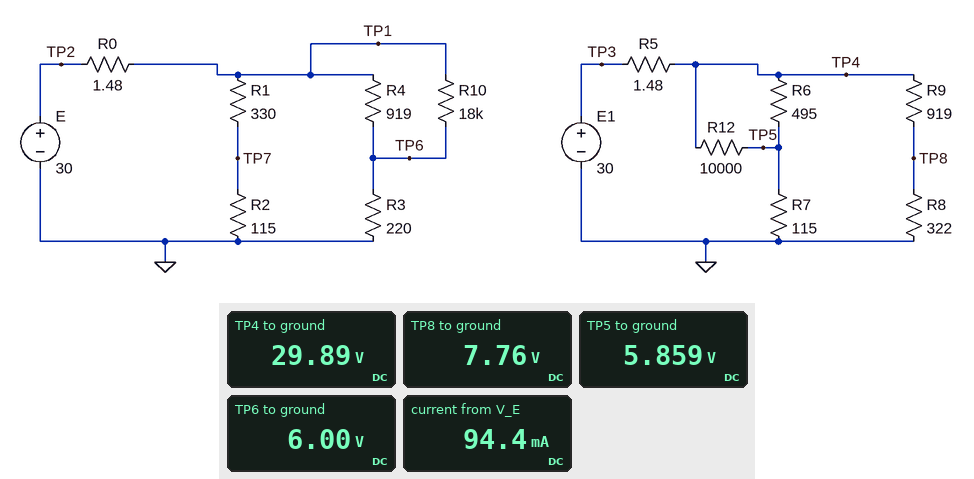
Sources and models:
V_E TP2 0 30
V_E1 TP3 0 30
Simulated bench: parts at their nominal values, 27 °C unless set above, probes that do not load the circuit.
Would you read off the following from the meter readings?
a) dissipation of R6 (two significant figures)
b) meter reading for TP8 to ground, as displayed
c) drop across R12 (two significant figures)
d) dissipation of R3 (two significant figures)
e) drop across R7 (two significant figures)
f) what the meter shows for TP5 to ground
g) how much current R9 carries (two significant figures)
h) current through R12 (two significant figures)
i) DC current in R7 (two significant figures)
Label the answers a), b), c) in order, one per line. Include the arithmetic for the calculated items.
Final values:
a) (29.89 V - 5.859 V)^2 / 495 Ω = 1.2 W
b) 7.76 V
c) 29.89 V - 5.859 V = 24 V
d) (6 V)^2 / 220 Ω = 160 mW
e) 5.859 V = 5.9 V
f) 5.859 V
g) (29.89 V - 7.76 V) / 919 Ω = 24 mA
h) (29.89 V - 5.859 V) / 10 kΩ = 2.4 mA
i) (5.859 V) / 115 Ω = 51 mA
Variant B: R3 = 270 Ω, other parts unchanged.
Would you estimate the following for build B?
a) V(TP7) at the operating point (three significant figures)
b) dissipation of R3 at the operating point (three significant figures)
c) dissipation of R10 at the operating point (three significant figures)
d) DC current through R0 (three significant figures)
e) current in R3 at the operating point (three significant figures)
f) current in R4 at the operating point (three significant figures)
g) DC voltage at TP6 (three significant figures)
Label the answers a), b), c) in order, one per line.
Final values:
a) 7.72 V
b) 184 mW
c) 28.9 mW
d) 93.2 mA
e) 26.1 mA
f) 24.8 mA
g) 7.05 V
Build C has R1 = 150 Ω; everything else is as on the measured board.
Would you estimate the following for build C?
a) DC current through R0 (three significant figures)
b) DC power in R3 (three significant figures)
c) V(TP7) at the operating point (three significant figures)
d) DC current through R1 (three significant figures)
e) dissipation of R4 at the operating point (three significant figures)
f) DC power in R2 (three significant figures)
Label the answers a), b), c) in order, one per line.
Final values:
a) 140 mA
b) 163 mW
c) 12.9 V
d) 112 mA
e) 617 mW
f) 1.45 W
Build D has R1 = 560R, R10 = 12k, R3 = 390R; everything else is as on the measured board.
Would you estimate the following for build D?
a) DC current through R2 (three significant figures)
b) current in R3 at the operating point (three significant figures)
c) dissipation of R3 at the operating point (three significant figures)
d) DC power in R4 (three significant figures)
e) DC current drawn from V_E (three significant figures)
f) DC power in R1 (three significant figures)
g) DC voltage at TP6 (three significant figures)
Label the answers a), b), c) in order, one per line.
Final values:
a) 44.3 mA
b) 24.0 mA
c) 225 mW
d) 458 mW
e) 68.3 mA
f) 1.10 W
g) 9.38 V
